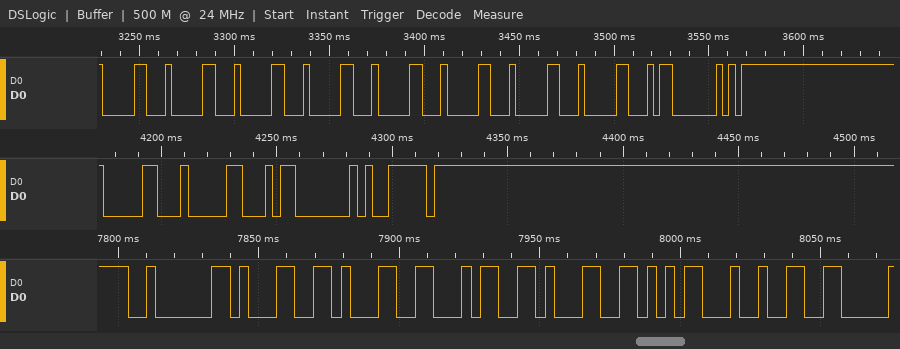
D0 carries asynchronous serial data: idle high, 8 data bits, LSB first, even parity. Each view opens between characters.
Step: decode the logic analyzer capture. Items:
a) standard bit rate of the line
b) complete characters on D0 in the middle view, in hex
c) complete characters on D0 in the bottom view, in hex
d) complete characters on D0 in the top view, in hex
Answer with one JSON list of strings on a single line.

["300 baud", "30, 30, 03, F9", "02, 31, 31, 34, 31, 35, 32", "30, 30, 30, 30, 30, 30, 30, 30, 03, FD"]
